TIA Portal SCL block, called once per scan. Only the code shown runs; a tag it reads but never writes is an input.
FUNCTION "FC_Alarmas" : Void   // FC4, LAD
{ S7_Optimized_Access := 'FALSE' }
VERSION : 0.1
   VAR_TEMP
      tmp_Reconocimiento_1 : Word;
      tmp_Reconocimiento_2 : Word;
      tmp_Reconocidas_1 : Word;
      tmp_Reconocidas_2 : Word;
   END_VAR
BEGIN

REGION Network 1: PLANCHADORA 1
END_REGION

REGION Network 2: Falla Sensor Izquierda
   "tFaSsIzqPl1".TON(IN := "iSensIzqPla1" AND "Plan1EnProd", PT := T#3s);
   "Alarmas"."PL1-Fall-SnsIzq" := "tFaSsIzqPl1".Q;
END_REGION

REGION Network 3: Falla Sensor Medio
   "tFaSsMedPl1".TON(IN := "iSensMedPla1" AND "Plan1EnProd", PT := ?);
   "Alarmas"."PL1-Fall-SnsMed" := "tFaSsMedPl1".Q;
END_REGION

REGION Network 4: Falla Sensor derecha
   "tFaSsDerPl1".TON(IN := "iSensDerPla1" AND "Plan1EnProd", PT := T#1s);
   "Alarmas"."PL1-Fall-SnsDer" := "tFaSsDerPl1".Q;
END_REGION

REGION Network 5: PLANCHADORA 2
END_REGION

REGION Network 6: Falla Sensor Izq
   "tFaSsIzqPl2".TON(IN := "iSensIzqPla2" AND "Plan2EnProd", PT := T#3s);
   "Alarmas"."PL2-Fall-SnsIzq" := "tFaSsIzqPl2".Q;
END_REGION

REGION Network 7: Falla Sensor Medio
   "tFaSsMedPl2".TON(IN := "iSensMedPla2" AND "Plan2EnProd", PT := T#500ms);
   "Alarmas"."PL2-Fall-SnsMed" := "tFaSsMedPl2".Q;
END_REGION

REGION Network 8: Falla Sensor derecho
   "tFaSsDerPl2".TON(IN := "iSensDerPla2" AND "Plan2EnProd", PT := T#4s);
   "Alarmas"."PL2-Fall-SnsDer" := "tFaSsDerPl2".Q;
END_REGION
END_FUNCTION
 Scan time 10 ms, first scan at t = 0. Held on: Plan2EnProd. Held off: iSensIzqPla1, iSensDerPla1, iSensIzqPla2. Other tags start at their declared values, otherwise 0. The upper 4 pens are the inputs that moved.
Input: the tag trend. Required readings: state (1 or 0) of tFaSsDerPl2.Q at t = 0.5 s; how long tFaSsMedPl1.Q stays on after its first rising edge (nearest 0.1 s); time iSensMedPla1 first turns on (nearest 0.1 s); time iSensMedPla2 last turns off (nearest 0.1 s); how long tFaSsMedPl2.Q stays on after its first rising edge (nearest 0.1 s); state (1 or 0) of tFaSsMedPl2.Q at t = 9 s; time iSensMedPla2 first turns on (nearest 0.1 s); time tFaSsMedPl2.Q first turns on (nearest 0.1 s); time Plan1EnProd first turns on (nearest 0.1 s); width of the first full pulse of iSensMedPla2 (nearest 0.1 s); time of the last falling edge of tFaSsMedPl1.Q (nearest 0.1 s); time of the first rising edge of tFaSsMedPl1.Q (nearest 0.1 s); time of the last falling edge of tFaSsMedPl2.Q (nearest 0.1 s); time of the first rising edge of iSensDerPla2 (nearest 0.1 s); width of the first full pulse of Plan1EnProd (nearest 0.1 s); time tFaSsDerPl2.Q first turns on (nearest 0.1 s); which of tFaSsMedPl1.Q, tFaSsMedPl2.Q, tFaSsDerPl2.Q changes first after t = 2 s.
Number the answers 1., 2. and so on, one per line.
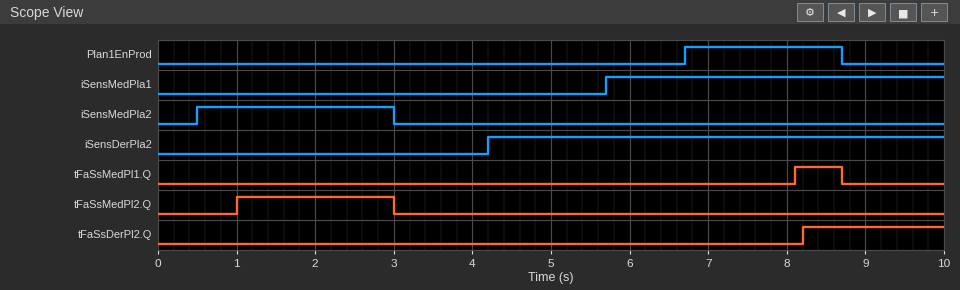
1. 0
2. 0.6 s
3. 5.7 s
4. 3.0 s
5. 2.0 s
6. 0
7. 0.5 s
8. 1.0 s
9. 6.7 s
10. 2.5 s
11. 8.7 s
12. 8.1 s
13. 3.0 s
14. 4.2 s
15. 2.0 s
16. 8.2 s
17. tFaSsMedPl2.Q
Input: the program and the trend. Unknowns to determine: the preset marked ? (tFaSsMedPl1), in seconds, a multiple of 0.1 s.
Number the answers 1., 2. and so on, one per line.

1. 1.4 s
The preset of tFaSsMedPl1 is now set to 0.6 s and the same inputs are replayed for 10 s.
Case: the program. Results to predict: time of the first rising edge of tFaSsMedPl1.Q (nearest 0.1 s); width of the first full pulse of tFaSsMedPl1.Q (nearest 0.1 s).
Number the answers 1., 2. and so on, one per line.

1. 7.3 s
2. 1.4 s
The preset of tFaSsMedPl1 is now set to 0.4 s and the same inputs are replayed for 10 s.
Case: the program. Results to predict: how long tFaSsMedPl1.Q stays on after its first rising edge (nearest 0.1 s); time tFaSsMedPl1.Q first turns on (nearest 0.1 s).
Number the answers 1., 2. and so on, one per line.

1. 1.6 s
2. 7.1 s
